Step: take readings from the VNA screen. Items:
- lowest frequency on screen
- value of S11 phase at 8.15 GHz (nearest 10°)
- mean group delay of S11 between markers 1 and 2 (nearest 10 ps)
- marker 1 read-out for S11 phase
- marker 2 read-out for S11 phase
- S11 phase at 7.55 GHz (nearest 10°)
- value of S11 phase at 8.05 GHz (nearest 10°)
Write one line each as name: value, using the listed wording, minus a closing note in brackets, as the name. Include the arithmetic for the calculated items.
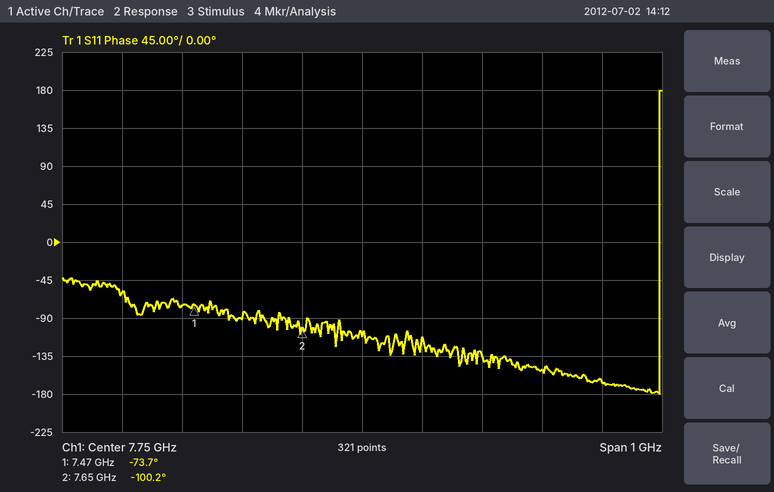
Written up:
lowest frequency on screen: 7.25 GHz
value of S11 phase at 8.15 GHz: -170°
mean group delay of S11 between markers 1 and 2: −(-100.2° − (-73.7°))/(360° × 180 MHz) ≈ 409 ps, so 410 ps to the nearest 10 ps
marker 1 read-out for S11 phase: -73.7°
marker 2 read-out for S11 phase: -100.2°
S11 phase at 7.55 GHz: -90°
value of S11 phase at 8.05 GHz: -150°
